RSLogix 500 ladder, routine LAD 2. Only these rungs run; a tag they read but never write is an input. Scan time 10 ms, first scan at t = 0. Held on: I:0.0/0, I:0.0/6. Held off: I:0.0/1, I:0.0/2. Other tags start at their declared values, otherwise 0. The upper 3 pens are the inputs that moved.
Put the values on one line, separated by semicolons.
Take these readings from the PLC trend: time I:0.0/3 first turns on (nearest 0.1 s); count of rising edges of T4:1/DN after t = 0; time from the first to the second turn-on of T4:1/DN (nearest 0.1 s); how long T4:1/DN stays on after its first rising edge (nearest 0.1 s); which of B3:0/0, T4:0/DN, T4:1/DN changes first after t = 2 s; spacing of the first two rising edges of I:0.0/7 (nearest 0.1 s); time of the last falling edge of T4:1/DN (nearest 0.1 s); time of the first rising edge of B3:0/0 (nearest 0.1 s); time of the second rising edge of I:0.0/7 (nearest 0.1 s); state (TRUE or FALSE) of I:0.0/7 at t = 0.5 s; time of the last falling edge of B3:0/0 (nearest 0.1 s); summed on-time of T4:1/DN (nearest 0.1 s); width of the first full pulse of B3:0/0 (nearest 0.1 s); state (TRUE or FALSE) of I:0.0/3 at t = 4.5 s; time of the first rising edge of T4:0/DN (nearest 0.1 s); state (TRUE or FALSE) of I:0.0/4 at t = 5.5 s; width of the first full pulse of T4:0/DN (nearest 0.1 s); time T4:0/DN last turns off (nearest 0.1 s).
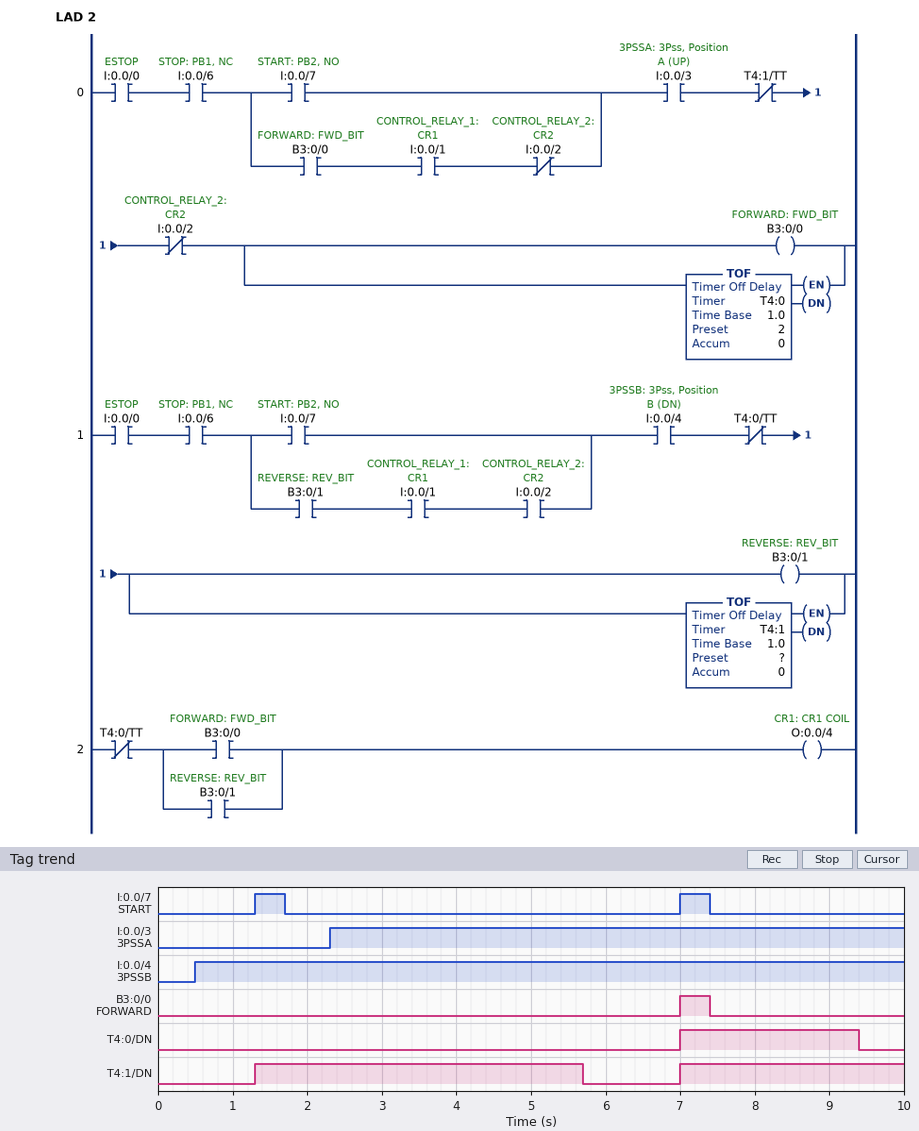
2.3 s; 2; 5.7 s; 4.4 s; T4:1/DN; 5.7 s; 5.7 s; 7.0 s; 7.0 s; FALSE; 7.4 s; 7.4 s; 0.4 s; TRUE; 7.0 s; TRUE; 2.4 s; 9.4 s
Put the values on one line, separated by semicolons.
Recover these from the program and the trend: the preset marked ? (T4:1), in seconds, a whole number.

4 s
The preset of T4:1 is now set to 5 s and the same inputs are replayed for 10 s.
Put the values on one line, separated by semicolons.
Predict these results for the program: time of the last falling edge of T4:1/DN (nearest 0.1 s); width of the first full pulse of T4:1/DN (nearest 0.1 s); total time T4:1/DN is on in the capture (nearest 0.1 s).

6.7 s; 5.4 s; 8.4 s
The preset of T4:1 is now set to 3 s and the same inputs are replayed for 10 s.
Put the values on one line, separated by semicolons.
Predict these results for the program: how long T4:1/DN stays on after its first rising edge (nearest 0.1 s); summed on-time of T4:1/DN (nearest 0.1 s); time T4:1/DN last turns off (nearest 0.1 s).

3.4 s; 6.4 s; 4.7 s
